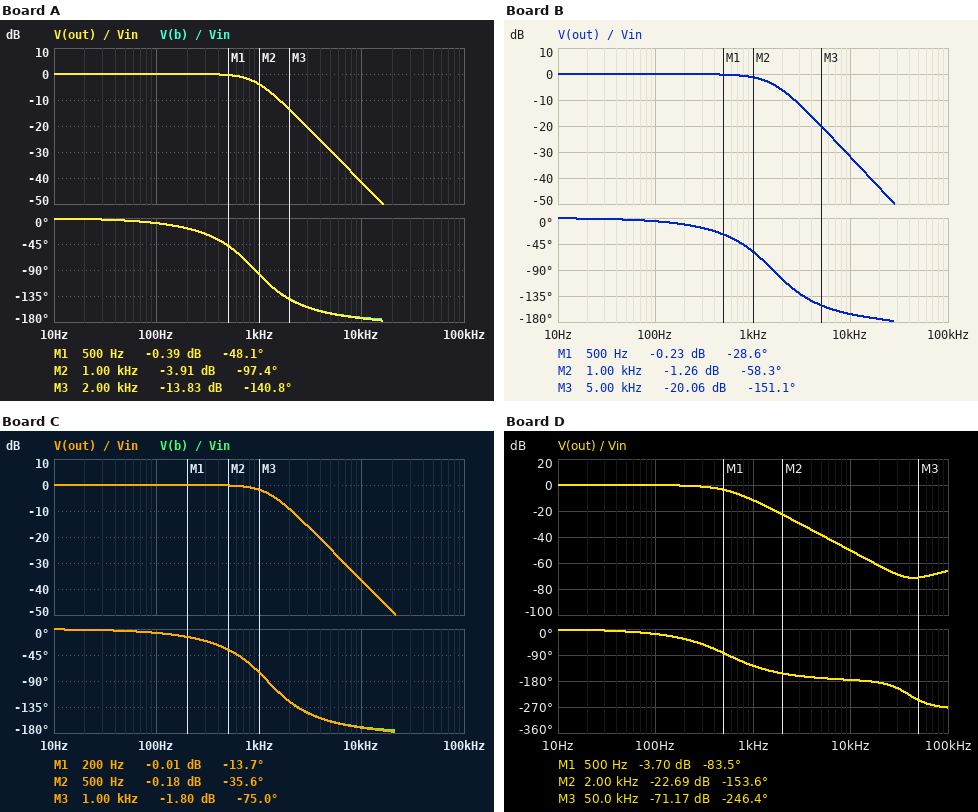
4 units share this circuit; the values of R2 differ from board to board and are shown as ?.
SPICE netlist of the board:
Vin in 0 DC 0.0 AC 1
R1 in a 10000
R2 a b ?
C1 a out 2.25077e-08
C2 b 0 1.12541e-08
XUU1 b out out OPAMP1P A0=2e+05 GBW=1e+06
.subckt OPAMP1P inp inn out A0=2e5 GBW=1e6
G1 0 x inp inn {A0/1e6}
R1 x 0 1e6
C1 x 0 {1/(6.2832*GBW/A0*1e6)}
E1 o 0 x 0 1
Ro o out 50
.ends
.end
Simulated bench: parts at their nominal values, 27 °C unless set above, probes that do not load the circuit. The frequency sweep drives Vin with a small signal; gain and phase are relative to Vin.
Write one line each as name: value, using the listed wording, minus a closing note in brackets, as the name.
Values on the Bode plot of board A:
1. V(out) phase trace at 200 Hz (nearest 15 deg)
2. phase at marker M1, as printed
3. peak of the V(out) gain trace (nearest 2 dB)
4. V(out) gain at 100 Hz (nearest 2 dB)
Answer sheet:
V(out) phase trace at 200 Hz: -15 deg
phase at marker M1, as printed: -48.1 deg
peak of the V(out) gain trace: 0 dB
V(out) gain at 100 Hz: 0 dB
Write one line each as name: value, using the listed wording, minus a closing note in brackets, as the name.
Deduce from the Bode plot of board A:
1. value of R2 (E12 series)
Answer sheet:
value of R2: 12 kΩ
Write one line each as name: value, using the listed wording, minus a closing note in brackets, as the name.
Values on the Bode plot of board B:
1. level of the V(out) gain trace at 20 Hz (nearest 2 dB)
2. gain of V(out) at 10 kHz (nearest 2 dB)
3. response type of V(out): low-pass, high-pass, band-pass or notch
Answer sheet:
level of the V(out) gain trace at 20 Hz: 0 dB
gain of V(out) at 10 kHz: -32 dB
response type of V(out): low-pass, high-pass, band-pass or notch: low-pass
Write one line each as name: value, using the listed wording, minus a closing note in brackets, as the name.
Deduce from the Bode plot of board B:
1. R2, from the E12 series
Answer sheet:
R2, from the E12 series: 3.9 kΩ
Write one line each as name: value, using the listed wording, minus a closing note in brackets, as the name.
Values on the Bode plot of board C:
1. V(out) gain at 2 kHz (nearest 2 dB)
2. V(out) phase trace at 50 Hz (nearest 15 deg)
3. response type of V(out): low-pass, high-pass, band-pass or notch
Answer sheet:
V(out) gain at 2 kHz: -10 dB
V(out) phase trace at 50 Hz: 0 deg
response type of V(out): low-pass, high-pass, band-pass or notch: low-pass
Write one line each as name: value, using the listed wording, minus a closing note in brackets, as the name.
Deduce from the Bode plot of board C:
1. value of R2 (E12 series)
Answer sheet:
value of R2: 6.8 kΩ
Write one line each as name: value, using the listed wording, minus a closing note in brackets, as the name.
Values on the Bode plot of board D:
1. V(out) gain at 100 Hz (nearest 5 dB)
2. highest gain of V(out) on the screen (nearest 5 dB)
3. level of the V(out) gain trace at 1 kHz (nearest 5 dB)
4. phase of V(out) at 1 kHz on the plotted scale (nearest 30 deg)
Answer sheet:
V(out) gain at 100 Hz: 0 dB
highest gain of V(out) on the screen: 0 dB
level of the V(out) gain trace at 1 kHz: -10 dB
phase of V(out) at 1 kHz on the plotted scale: -120 deg
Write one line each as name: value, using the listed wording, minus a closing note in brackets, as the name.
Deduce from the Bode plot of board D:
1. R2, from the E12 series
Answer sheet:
R2, from the E12 series: 33 kΩ
